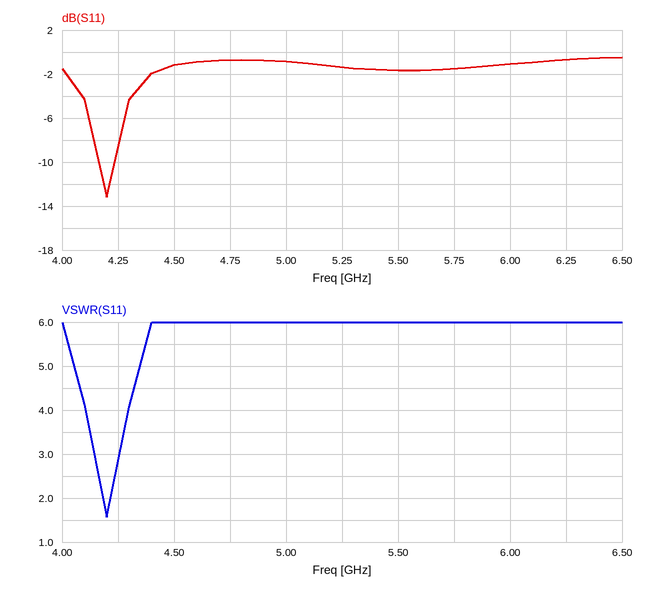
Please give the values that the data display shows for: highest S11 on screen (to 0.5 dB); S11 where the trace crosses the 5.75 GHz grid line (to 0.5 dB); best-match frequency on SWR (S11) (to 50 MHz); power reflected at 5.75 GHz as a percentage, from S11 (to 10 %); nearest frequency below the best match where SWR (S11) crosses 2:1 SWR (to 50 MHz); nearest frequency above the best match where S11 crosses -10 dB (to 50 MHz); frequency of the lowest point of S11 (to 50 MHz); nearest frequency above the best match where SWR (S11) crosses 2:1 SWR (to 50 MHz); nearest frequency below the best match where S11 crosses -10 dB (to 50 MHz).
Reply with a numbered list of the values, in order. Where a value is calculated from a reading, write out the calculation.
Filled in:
1. -0.5 dB
2. -1.5 dB
3. 4.20 GHz
4. 10^(-1.5/10) ≈ 70.8 %, so 70 % to the nearest 10 %
5. 4.20 GHz
6. 4.25 GHz
7. 4.20 GHz
8. 4.20 GHz
9. 4.15 GHz
